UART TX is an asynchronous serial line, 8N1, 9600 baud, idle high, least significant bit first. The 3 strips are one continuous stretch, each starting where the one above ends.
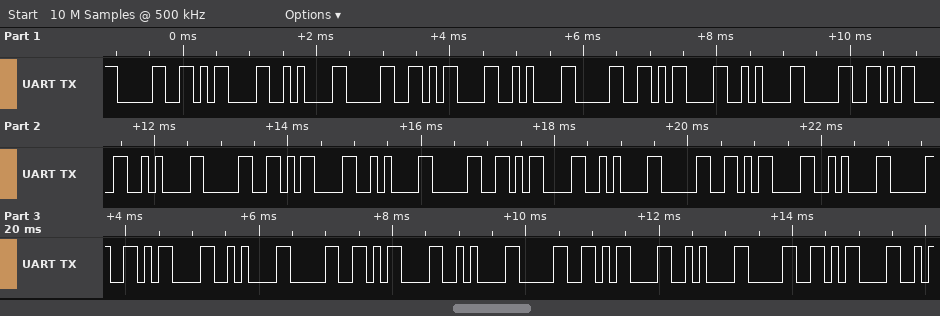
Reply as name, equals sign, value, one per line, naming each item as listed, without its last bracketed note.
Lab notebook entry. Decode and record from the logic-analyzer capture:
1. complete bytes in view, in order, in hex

complete bytes in view, in order, in hex = 0x30 0x0D 0x0A 0x30 0x0D 0x0A 0x30 0x0D 0x0A 0x30 0x0D 0x0A 0x30 0x0D 0x0A 0x30 0x0D 0x0A 0x30 0x0D 0x0A 0x30 0x0D 0x0A 0x30 0x0D 0x0A 0x30 0x0D 0x0A 0x30 0x0D
